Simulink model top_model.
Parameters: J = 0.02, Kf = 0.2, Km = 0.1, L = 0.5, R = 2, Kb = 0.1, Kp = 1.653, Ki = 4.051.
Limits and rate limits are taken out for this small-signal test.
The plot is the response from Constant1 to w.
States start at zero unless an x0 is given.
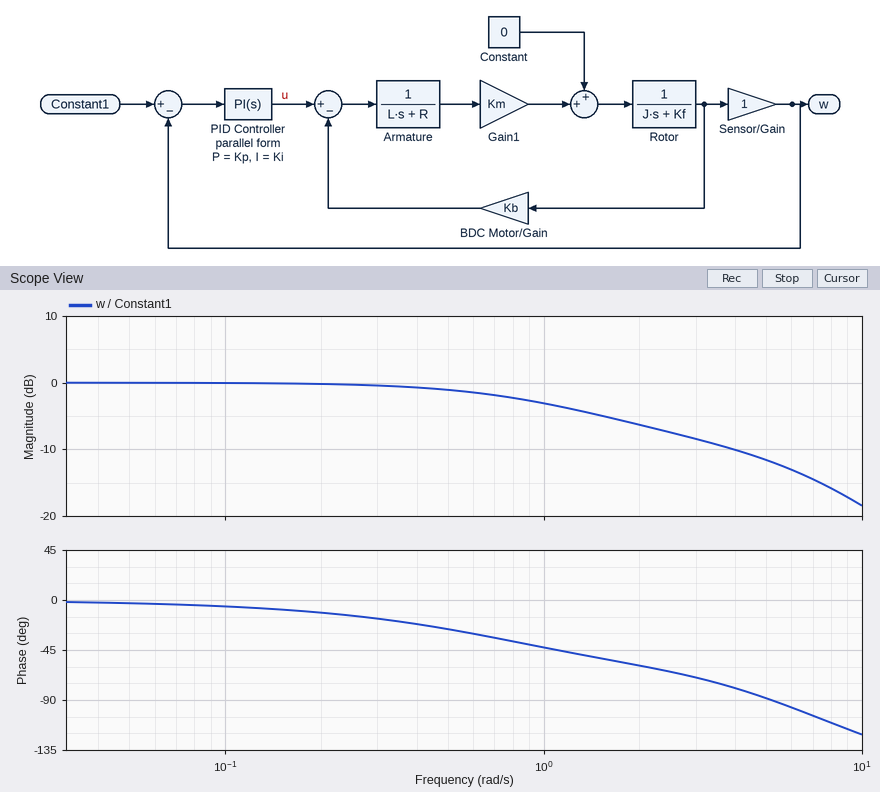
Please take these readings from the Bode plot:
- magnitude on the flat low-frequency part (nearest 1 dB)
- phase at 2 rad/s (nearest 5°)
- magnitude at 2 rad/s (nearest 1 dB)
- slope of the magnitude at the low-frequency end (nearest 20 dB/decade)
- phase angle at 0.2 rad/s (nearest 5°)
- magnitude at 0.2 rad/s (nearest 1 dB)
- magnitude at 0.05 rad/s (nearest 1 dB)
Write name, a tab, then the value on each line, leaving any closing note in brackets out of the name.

magnitude on the flat low-frequency part	0 dB
phase at 2 rad/s	-60°
magnitude at 2 rad/s	-6 dB
slope of the magnitude at the low-frequency end	0 dB/decade
phase angle at 0.2 rad/s	-10°
magnitude at 0.2 rad/s	0 dB
magnitude at 0.05 rad/s	0 dB
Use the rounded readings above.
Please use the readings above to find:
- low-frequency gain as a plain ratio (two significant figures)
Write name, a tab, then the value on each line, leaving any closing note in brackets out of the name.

low-frequency gain as a plain ratio	1.0
